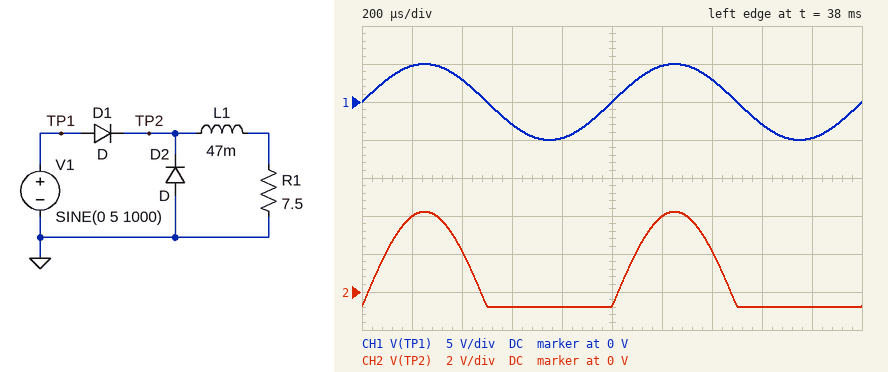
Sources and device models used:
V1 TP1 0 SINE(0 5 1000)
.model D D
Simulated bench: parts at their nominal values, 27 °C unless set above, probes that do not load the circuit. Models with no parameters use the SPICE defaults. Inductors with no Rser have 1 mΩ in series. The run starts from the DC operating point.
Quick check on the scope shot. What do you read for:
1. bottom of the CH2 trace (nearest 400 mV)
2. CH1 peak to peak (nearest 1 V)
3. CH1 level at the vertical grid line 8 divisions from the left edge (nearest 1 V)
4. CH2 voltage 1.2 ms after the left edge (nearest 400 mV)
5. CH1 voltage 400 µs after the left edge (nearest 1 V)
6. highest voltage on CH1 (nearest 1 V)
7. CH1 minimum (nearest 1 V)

-800 mV
10 V
-3 V
4.0 V
3 V
5 V
-5 V
